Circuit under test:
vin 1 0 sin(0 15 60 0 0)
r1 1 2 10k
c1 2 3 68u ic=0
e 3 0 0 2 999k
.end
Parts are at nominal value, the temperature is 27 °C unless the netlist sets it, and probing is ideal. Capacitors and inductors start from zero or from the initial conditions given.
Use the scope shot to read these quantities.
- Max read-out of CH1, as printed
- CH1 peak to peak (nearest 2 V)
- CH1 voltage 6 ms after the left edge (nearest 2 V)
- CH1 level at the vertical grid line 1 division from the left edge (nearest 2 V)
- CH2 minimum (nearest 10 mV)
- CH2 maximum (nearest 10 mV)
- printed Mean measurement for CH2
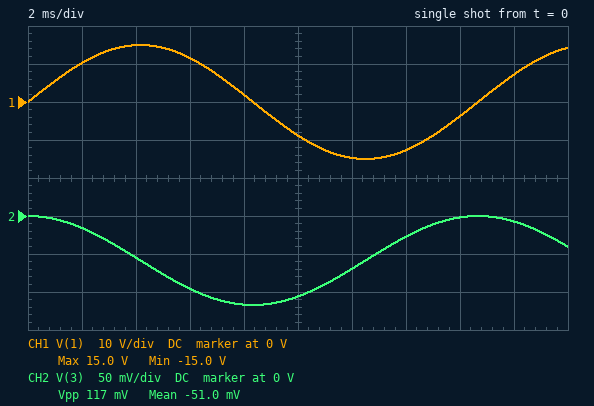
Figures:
15.0 V
30 V
12 V
10 V
-120 mV
0 V
-51.0 mV
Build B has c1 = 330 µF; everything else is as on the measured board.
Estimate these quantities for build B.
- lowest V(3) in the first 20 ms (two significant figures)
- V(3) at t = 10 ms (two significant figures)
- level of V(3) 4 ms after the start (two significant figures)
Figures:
-24 mV
-22 mV
-11 mV
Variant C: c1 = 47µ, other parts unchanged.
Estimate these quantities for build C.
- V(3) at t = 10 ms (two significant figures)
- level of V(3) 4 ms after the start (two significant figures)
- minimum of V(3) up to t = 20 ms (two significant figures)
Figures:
-150 mV
-79 mV
-170 mV
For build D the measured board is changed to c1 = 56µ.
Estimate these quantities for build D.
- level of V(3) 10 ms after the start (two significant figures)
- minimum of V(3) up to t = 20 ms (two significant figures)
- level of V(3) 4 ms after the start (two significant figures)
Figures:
-130 mV
-140 mV
-67 mV
